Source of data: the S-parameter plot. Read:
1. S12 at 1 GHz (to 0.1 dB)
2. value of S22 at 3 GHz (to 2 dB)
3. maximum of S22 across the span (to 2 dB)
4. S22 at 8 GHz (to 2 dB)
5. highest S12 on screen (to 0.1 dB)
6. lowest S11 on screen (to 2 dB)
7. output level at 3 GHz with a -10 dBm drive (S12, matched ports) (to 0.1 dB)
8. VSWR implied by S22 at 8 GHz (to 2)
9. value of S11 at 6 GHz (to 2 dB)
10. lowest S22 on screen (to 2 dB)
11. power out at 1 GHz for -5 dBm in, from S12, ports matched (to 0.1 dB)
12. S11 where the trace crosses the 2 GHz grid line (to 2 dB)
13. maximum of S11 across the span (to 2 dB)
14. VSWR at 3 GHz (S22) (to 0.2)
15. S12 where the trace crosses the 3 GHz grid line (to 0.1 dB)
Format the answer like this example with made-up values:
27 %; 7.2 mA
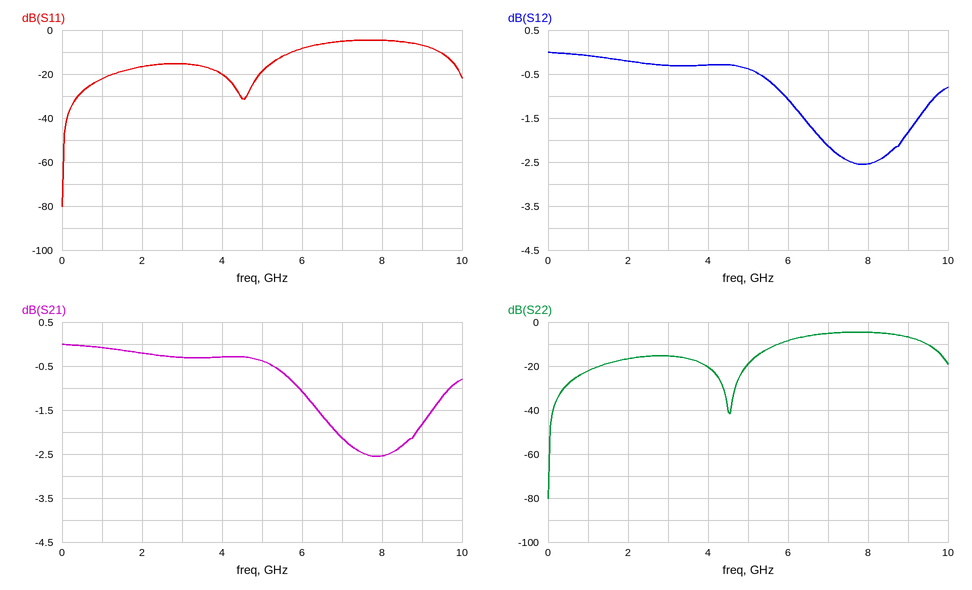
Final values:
-0.1 dB; -16 dB; -4 dB; -4 dB; 0.0 dB; -80 dB; -10.3 dBm; 4; -8 dB; -80 dB; -5.1 dBm; -16 dB; -4 dB; 1.4; -0.3 dB
